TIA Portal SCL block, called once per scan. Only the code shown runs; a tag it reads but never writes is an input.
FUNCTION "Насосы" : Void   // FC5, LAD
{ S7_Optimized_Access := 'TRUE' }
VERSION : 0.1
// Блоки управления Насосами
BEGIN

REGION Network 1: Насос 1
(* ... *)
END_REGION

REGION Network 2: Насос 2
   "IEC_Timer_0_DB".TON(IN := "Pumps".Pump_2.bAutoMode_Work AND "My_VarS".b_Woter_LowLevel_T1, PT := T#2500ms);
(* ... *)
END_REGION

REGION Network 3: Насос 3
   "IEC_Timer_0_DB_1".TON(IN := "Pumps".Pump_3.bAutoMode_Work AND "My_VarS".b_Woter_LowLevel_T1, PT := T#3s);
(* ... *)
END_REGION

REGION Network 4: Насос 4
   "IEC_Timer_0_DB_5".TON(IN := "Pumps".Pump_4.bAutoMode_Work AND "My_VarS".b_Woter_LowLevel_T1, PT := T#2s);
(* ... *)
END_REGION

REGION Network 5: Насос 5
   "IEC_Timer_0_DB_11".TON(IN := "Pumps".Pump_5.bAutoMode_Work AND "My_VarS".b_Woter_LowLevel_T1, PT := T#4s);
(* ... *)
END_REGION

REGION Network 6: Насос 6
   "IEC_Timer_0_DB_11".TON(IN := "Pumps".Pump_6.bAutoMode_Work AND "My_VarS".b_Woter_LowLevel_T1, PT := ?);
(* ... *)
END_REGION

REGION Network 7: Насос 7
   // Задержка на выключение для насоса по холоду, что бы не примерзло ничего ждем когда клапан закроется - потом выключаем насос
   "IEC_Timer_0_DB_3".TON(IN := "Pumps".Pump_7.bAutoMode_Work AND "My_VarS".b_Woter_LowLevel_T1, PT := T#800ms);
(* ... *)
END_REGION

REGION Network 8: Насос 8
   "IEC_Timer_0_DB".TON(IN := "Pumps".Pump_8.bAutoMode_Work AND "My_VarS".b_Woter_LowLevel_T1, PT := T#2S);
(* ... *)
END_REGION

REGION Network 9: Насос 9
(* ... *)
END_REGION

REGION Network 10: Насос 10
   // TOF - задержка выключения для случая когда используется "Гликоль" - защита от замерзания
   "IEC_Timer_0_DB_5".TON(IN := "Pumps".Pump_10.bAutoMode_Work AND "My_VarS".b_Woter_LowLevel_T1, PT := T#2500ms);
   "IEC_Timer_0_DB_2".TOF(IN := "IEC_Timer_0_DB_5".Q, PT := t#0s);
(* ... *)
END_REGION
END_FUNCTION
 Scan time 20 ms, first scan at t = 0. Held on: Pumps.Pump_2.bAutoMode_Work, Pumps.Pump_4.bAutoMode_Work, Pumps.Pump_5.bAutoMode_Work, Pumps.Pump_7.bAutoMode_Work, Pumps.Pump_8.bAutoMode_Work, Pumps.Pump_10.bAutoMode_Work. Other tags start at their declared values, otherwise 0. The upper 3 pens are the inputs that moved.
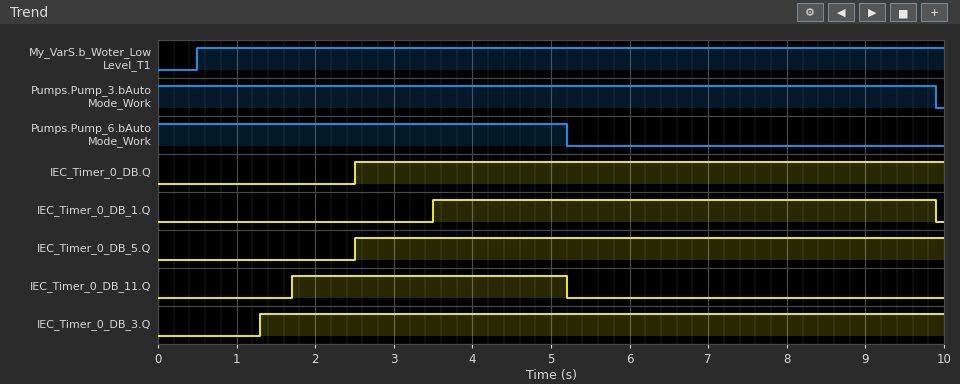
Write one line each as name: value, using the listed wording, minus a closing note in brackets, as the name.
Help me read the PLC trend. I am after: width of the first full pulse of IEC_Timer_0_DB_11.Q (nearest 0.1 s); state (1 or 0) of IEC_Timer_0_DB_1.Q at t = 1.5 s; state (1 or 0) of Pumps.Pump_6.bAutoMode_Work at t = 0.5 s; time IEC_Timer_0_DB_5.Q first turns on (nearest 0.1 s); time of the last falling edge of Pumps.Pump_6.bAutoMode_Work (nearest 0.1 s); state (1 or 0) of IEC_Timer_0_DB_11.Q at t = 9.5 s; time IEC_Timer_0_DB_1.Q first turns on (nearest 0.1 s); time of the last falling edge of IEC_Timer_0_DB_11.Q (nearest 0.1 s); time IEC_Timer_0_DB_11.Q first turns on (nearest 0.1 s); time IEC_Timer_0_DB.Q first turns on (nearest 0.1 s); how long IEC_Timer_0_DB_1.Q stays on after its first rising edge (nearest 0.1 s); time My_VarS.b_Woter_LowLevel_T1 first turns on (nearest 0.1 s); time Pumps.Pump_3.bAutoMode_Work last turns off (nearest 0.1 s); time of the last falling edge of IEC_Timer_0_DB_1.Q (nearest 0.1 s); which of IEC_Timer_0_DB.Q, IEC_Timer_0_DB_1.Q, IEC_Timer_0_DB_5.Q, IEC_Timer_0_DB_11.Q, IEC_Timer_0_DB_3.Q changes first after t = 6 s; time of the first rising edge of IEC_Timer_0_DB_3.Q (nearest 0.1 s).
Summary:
width of the first full pulse of IEC_Timer_0_DB_11.Q: 3.5 s
state (1 or 0) of IEC_Timer_0_DB_1.Q at t = 1.5 s: 0
state (1 or 0) of Pumps.Pump_6.bAutoMode_Work at t = 0.5 s: 1
time IEC_Timer_0_DB_5.Q first turns on: 2.5 s
time of the last falling edge of Pumps.Pump_6.bAutoMode_Work: 5.2 s
state (1 or 0) of IEC_Timer_0_DB_11.Q at t = 9.5 s: 0
time IEC_Timer_0_DB_1.Q first turns on: 3.5 s
time of the last falling edge of IEC_Timer_0_DB_11.Q: 5.2 s
time IEC_Timer_0_DB_11.Q first turns on: 1.7 s
time IEC_Timer_0_DB.Q first turns on: 2.5 s
how long IEC_Timer_0_DB_1.Q stays on after its first rising edge: 6.4 s
time My_VarS.b_Woter_LowLevel_T1 first turns on: 0.5 s
time Pumps.Pump_3.bAutoMode_Work last turns off: 9.9 s
time of the last falling edge of IEC_Timer_0_DB_1.Q: 9.9 s
which of IEC_Timer_0_DB.Q, IEC_Timer_0_DB_1.Q, IEC_Timer_0_DB_5.Q, IEC_Timer_0_DB_11.Q, IEC_Timer_0_DB_3.Q changes first after t = 6 s: IEC_Timer_0_DB_1.Q
time of the first rising edge of IEC_Timer_0_DB_3.Q: 1.3 s
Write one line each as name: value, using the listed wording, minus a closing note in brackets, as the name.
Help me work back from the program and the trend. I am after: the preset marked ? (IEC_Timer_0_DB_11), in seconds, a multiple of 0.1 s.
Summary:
the preset marked ? (IEC_Timer_0_DB_11), in seconds, a multiple of 0.1 s: 1.2 s
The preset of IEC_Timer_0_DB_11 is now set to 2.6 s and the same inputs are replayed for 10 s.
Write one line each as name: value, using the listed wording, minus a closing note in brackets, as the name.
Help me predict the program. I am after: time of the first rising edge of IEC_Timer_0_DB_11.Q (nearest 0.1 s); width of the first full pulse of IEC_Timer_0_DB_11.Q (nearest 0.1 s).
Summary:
time of the first rising edge of IEC_Timer_0_DB_11.Q: 3.1 s
width of the first full pulse of IEC_Timer_0_DB_11.Q: 2.1 s
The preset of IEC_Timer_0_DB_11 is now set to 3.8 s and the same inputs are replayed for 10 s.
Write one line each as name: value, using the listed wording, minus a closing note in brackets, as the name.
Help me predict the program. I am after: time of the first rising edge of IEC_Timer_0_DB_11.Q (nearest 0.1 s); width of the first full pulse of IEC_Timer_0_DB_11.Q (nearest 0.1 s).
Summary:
time of the first rising edge of IEC_Timer_0_DB_11.Q: 4.3 s
width of the first full pulse of IEC_Timer_0_DB_11.Q: 0.9 s
